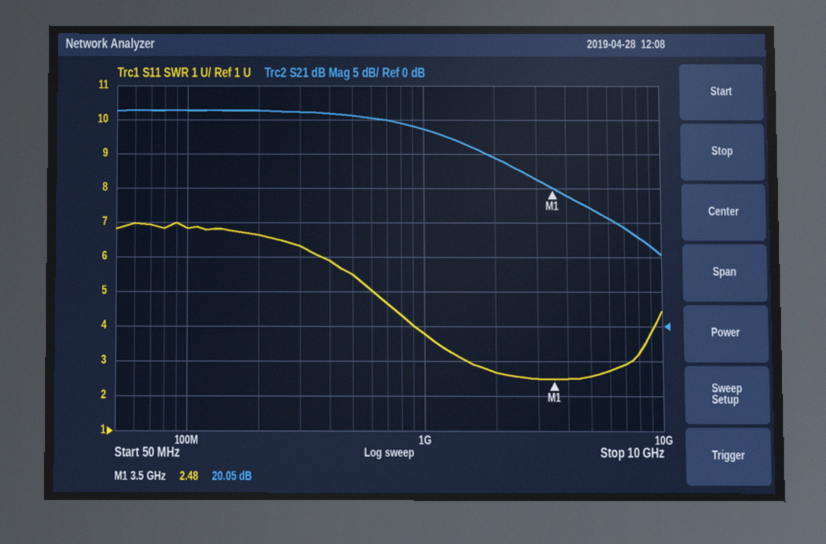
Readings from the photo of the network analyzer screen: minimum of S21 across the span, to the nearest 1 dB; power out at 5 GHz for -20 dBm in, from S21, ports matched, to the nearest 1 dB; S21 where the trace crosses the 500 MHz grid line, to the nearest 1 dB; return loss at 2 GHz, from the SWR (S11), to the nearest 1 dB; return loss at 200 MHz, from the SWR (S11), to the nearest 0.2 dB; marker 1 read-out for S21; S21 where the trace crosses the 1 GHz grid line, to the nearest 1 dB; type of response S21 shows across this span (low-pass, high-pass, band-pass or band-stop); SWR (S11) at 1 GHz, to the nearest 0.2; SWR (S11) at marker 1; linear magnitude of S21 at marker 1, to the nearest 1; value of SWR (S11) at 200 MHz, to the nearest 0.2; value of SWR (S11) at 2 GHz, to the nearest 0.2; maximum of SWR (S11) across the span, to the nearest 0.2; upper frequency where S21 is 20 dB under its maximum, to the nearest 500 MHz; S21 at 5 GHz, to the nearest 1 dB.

10 dB
-3 dBm
31 dB
7 dB
2.6 dB
20.05 dB
29 dB
low-pass
3.8
2.48
10
6.6
2.6
7.0
9.0 GHz
17 dB
